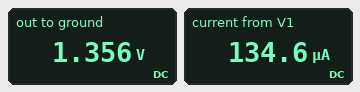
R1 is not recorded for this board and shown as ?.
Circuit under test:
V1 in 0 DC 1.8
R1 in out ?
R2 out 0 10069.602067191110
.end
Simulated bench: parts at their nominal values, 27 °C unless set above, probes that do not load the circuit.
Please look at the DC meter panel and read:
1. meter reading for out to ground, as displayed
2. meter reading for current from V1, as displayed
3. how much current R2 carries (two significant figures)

1.356 V
134.6 µA
130 µA
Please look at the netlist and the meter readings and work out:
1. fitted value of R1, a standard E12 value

3.3 kΩ
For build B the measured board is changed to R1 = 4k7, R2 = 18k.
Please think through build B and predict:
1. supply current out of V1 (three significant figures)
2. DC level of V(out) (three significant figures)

79.3 µA
1.43 V
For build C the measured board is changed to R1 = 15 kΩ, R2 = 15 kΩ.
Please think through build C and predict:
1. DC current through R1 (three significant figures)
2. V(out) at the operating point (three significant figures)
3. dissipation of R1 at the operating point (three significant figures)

60.0 µA
900 mV
54.0 µW
